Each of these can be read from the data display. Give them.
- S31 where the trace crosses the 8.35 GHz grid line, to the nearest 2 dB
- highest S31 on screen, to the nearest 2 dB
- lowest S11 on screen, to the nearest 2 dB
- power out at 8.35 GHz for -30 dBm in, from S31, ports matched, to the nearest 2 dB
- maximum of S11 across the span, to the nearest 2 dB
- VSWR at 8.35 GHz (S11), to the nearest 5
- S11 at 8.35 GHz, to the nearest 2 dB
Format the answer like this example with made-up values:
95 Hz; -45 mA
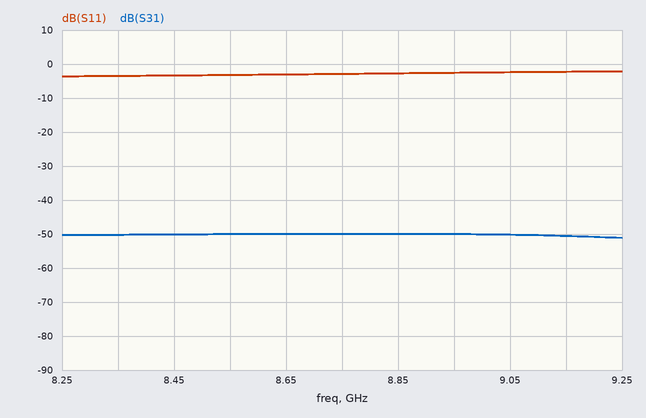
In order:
-50 dB; -50 dB; -4 dB; -80 dBm; -2 dB; 5; -4 dB
